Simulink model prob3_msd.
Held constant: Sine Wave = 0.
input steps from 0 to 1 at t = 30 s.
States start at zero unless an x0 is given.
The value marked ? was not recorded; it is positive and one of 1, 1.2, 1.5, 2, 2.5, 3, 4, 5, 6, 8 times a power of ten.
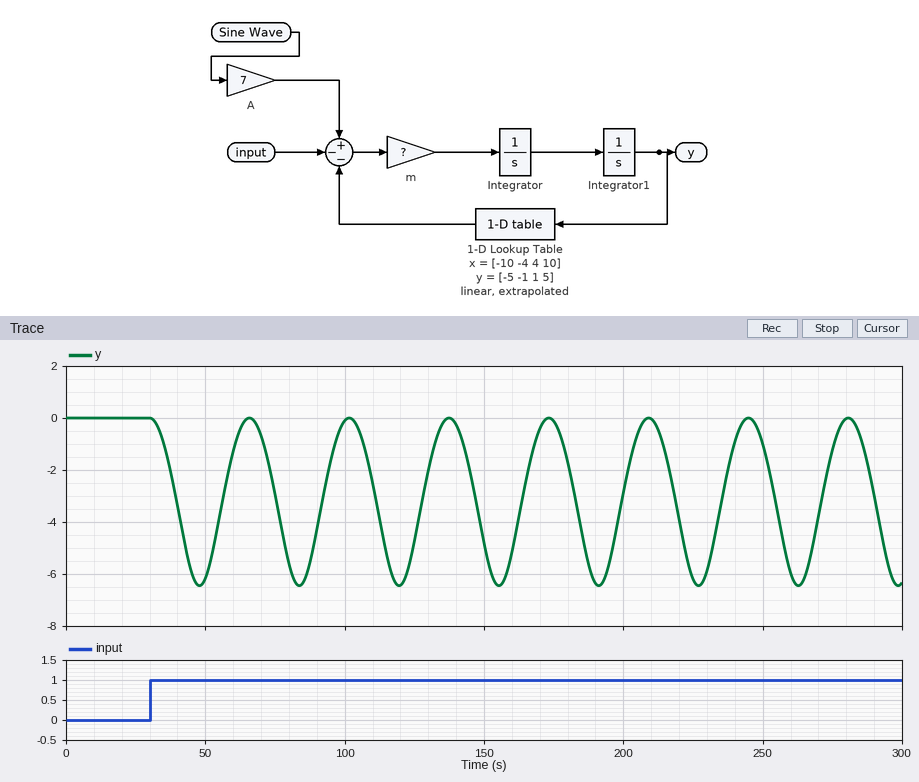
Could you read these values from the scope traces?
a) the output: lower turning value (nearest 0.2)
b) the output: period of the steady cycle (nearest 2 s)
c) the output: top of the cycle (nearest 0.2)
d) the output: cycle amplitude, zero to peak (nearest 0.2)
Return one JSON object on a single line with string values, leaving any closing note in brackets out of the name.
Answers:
{"the output: lower turning value": "-6.4", "the output: period of the steady cycle": "36 s", "the output: top of the cycle": "0.0", "the output: cycle amplitude, zero to peak": "3.2"}
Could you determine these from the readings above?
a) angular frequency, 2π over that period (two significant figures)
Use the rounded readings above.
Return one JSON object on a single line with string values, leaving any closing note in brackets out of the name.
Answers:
{"angular frequency, 2π over that period": "0.17 rad/s"}
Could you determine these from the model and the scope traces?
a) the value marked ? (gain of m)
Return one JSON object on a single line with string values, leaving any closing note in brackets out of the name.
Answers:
{"the value marked ?": "0.08"}
